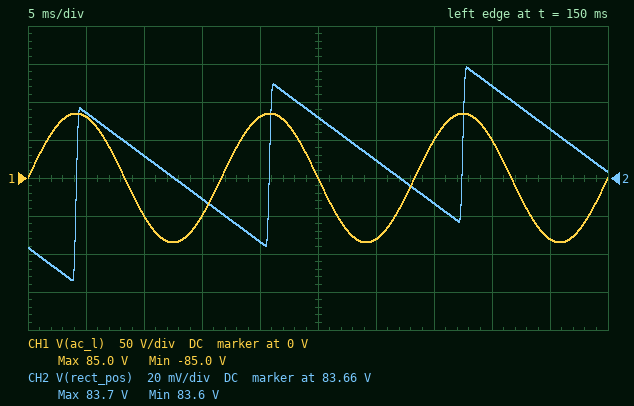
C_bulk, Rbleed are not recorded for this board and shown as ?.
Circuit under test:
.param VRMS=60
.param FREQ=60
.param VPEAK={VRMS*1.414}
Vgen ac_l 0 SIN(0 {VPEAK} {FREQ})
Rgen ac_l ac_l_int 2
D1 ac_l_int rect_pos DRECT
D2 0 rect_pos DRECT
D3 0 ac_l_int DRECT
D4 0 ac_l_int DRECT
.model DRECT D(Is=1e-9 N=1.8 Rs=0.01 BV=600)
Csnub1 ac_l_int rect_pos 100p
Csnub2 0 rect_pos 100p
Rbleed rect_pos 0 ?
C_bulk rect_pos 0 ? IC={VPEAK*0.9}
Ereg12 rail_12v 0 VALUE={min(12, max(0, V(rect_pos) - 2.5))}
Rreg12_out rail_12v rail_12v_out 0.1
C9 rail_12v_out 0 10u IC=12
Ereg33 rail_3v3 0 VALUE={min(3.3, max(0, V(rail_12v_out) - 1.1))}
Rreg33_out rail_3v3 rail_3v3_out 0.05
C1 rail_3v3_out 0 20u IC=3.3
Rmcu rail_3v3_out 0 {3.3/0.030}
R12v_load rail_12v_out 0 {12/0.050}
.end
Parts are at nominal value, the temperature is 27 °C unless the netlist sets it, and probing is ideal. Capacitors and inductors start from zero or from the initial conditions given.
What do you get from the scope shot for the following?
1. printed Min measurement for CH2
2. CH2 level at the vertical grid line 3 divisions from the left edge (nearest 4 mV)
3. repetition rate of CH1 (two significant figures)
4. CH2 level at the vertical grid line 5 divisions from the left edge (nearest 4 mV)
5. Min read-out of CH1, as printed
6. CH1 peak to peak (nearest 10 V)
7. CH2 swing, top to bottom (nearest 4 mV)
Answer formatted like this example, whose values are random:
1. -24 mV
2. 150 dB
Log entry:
1. 83.6 V
2. 83.648 V
3. 60 Hz
4. 83.692 V
5. -85.0 V
6. 170 V
7. 112 mV
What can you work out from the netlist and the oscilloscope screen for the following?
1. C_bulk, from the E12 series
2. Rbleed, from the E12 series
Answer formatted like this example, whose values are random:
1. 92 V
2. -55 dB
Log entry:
1. 560 µF
2. 33 kΩ
